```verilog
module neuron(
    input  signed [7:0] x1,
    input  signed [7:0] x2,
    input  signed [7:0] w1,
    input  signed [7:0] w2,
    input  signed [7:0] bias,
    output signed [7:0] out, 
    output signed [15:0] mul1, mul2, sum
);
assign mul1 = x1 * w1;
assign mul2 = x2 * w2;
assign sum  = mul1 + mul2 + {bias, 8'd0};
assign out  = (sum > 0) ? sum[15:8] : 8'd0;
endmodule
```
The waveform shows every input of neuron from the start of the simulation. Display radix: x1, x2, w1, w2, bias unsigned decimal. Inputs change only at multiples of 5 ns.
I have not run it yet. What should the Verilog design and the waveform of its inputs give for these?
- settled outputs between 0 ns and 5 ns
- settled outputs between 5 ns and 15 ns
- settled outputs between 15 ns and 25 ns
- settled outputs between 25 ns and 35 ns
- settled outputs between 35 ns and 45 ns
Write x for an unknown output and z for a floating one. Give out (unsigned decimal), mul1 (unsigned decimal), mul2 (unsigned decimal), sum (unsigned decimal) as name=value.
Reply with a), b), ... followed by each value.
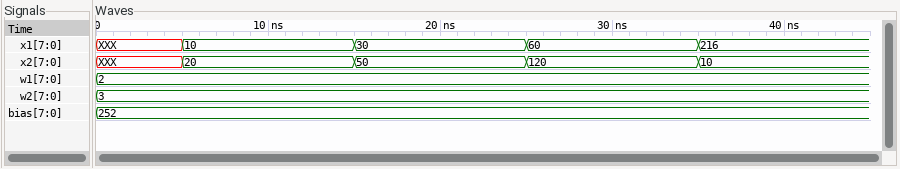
a) out=x, mul1=x, mul2=x, sum=x
b) out=0, mul1=20, mul2=60, sum=64592
c) out=0, mul1=60, mul2=150, sum=64722
d) out=0, mul1=120, mul2=360, sum=64992
e) out=0, mul1=65456, mul2=30, sum=64462
